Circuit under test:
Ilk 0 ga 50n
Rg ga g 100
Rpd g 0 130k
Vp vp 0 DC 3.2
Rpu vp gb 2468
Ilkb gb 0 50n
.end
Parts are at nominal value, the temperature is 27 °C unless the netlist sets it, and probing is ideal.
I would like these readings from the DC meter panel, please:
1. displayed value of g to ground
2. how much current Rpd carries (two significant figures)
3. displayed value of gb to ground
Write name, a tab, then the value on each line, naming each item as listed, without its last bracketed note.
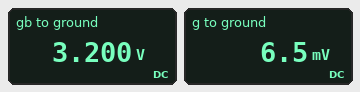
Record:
displayed value of g to ground	6.5 mV
how much current Rpd carries	50 nA
displayed value of gb to ground	3.200 V
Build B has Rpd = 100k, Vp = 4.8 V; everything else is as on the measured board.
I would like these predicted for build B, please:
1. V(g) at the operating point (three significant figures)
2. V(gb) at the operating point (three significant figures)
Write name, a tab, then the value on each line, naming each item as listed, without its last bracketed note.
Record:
V(g) at the operating point	5.00 mV
V(gb) at the operating point	4.80 V
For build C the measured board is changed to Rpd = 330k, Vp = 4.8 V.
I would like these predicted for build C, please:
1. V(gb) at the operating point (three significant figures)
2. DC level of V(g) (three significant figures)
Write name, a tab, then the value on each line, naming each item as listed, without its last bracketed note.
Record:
V(gb) at the operating point	4.80 V
DC level of V(g)	16.5 mV
